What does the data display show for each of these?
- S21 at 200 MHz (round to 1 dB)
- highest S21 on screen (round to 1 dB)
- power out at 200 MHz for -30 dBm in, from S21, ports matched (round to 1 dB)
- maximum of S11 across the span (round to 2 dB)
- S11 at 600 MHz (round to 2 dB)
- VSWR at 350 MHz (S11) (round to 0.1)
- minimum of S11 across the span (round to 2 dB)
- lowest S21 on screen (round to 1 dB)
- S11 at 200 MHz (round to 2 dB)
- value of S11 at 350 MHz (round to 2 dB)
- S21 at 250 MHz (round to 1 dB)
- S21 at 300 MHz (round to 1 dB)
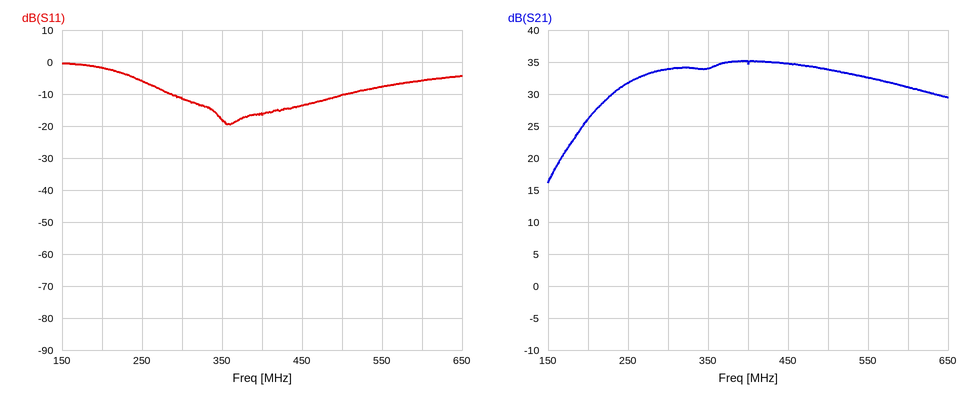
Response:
26 dB
35 dB
-4 dBm
0 dB
-6 dB
1.3
-20 dB
16 dB
-2 dB
-18 dB
32 dB
34 dB
